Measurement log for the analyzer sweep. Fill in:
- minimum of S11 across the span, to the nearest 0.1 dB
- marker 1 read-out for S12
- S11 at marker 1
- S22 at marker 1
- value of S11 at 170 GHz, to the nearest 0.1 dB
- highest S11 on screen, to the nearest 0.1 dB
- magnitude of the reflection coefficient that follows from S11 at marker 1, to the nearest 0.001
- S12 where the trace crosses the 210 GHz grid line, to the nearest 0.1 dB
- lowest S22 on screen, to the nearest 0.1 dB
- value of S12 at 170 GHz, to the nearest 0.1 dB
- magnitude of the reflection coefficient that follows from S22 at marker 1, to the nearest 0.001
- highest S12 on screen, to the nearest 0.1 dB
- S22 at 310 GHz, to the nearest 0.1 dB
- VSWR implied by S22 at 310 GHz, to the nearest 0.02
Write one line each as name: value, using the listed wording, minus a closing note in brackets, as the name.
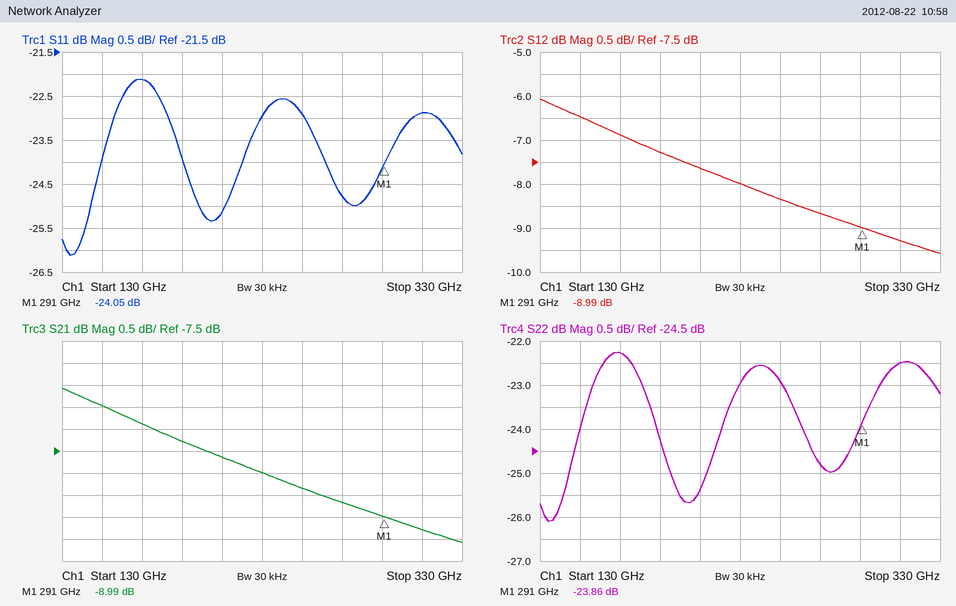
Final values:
minimum of S11 across the span, to the nearest 0.1 dB: -26.1 dB
marker 1 read-out for S12: -8.99 dB
S11 at marker 1: -24.05 dB
S22 at marker 1: -23.86 dB
value of S11 at 170 GHz, to the nearest 0.1 dB: -22.1 dB
highest S11 on screen, to the nearest 0.1 dB: -22.1 dB
magnitude of the reflection coefficient that follows from S11 at marker 1, to the nearest 0.001: 0.063
S12 where the trace crosses the 210 GHz grid line, to the nearest 0.1 dB: -7.6 dB
lowest S22 on screen, to the nearest 0.1 dB: -26.1 dB
value of S12 at 170 GHz, to the nearest 0.1 dB: -6.9 dB
magnitude of the reflection coefficient that follows from S22 at marker 1, to the nearest 0.001: 0.064
highest S12 on screen, to the nearest 0.1 dB: -6.1 dB
S22 at 310 GHz, to the nearest 0.1 dB: -22.5 dB
VSWR implied by S22 at 310 GHz, to the nearest 0.02: 1.16
